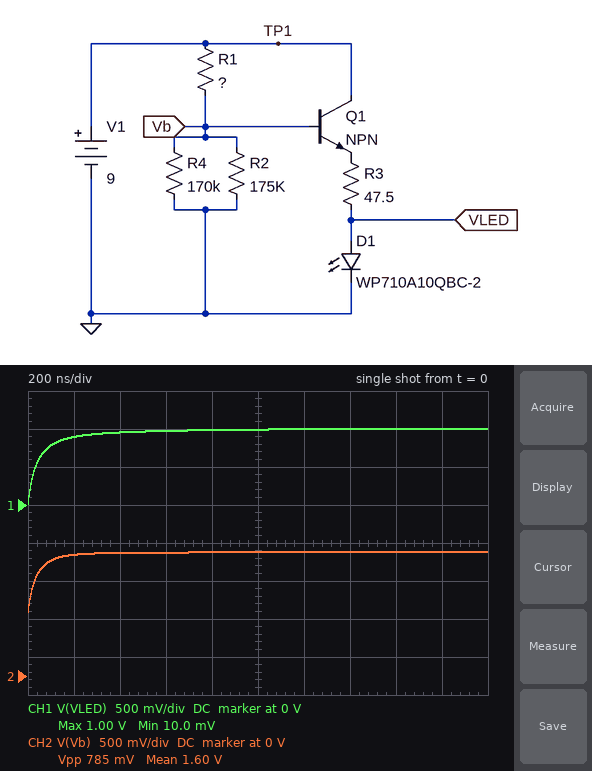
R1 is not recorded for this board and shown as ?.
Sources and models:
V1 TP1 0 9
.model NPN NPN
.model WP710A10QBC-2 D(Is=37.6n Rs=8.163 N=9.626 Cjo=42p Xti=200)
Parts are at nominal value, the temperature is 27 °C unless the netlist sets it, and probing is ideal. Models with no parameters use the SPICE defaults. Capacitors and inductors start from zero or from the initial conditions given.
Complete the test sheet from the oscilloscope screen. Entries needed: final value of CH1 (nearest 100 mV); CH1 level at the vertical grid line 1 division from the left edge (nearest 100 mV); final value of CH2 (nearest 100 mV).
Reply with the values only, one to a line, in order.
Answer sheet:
1.0 V
900 mV
1.6 V
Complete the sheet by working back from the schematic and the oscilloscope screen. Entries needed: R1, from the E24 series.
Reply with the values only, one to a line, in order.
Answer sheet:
390 kΩ
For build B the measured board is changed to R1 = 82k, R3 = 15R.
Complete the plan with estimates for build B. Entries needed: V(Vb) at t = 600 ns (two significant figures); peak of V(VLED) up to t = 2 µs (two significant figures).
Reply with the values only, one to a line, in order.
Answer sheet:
3.6 V
2.8 V
